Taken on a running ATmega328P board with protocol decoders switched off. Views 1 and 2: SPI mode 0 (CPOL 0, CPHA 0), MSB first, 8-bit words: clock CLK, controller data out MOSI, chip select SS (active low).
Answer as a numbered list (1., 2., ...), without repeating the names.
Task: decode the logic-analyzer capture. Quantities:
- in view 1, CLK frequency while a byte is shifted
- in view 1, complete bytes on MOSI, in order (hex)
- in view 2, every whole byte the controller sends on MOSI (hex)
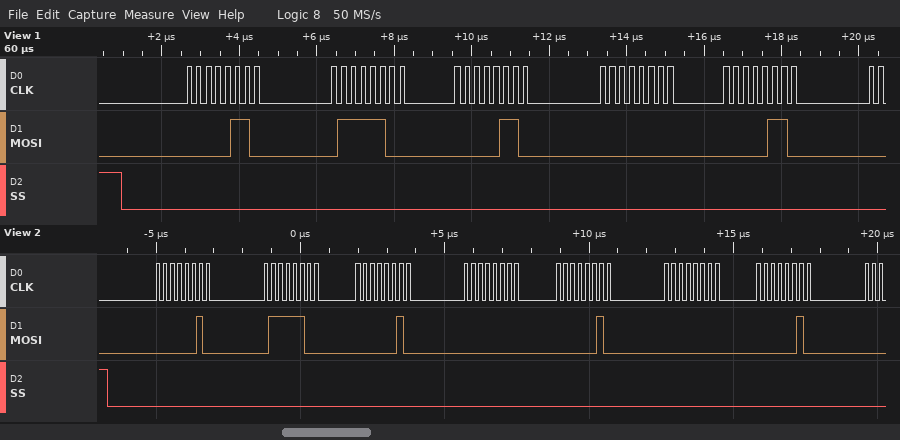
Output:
1. 4 MHz
2. 06 7C 06 00 06
3. 02 7C 02 00 02 00 02
